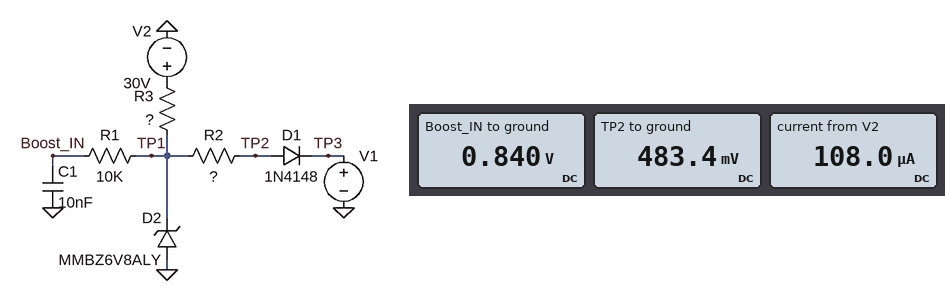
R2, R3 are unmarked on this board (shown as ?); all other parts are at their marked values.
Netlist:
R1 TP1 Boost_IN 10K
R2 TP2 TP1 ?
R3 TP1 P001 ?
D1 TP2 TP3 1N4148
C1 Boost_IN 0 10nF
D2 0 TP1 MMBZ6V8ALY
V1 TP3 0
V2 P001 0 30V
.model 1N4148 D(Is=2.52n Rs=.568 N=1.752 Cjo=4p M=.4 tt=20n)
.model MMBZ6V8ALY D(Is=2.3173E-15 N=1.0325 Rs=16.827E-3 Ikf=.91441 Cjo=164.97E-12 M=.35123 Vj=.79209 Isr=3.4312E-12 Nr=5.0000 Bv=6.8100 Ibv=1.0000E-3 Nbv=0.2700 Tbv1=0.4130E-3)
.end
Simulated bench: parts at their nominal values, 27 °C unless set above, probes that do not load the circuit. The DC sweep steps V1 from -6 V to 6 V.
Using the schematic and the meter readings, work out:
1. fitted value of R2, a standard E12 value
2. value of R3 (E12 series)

3.3 kΩ
270 kΩ
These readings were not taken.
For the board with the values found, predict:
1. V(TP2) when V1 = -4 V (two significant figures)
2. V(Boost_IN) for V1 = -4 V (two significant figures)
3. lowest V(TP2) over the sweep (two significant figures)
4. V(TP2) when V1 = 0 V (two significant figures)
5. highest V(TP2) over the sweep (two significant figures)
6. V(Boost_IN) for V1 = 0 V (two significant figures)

-3.4 V
-710 mV
-5.4 V
480 mV
6.5 V
840 mV
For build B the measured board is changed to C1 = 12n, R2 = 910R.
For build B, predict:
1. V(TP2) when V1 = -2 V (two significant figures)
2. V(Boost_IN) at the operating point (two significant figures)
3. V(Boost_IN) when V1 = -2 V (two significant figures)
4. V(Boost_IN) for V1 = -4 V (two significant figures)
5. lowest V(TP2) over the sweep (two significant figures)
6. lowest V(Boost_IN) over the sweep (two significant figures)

-1.4 V
580 mV
-710 mV
-740 mV
-5.3 V
-760 mV
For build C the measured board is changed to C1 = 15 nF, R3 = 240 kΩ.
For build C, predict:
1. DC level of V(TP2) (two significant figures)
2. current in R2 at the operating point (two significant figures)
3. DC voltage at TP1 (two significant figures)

490 mV
120 µA
890 mV
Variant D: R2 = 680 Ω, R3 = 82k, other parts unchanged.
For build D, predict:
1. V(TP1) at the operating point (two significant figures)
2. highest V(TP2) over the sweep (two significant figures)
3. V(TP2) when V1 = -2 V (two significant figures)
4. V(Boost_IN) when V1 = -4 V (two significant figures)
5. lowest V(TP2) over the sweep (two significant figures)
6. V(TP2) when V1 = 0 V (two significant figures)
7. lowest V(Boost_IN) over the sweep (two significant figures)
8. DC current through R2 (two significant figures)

780 mV
6.5 V
-1.4 V
-750 mV
-5.3 V
540 mV
-770 mV
360 µA
